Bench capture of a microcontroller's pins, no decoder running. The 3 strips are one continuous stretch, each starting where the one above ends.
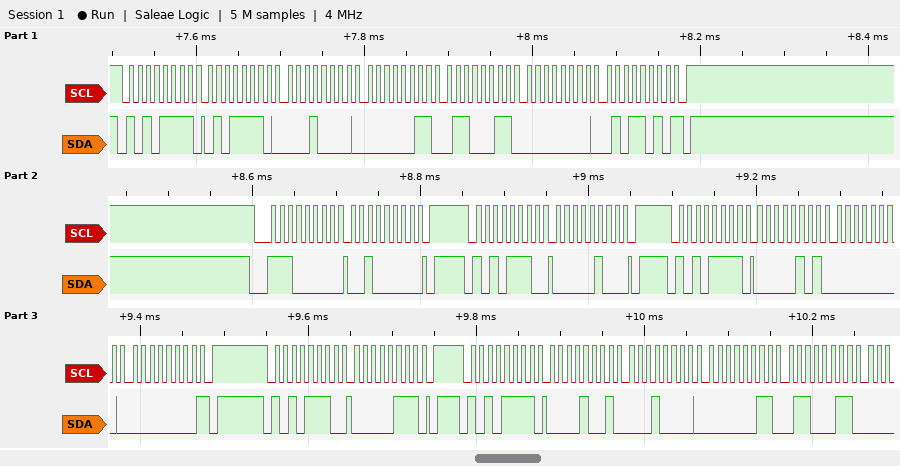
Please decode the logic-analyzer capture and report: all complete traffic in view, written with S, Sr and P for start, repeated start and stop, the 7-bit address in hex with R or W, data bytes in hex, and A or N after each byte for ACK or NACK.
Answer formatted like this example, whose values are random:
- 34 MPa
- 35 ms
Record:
- S 57R A 5E A 10 A 03 A 63 A 00 A 5A N P S 70W A 20 A P S 57W A 04 A P S 57R A 05 A 00 A 00 N P S 57W A 07 A P S 57R A 09 A 10 A 03 A 63 A
